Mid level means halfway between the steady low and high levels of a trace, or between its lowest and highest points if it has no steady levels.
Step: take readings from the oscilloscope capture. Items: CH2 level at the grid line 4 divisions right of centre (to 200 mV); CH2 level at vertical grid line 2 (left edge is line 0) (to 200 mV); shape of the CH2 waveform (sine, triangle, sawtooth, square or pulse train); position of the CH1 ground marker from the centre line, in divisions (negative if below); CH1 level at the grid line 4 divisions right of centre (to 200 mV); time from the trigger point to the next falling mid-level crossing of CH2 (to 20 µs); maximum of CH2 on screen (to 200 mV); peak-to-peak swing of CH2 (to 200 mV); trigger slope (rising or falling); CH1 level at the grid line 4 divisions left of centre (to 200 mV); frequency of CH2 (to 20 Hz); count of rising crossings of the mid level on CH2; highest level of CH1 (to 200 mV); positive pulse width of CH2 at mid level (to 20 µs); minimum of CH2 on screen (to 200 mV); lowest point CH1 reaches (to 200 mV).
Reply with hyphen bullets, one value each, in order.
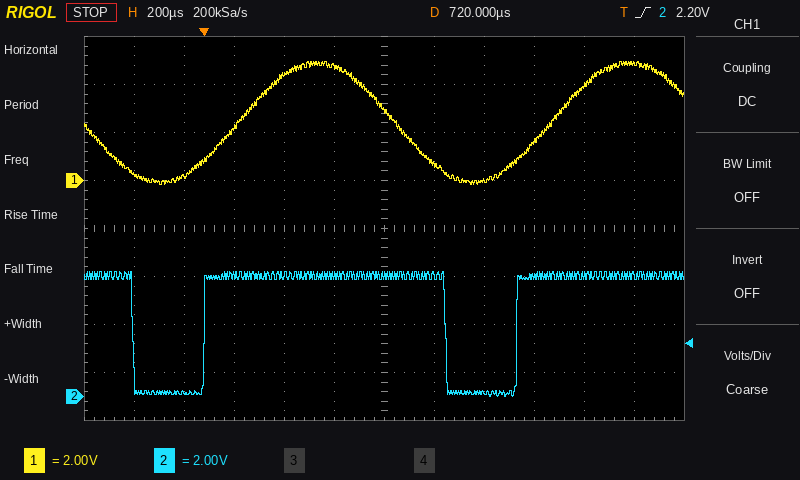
- 5.0 V
- 200 mV
- pulse train
- +1.0 div
- 4.0 V
- 960 µs
- 5.2 V
- 5.2 V
- rising
- 200 mV
- 800 Hz
- 2
- 5.0 V
- 960 µs
- 0.0 V
- -200 mV
